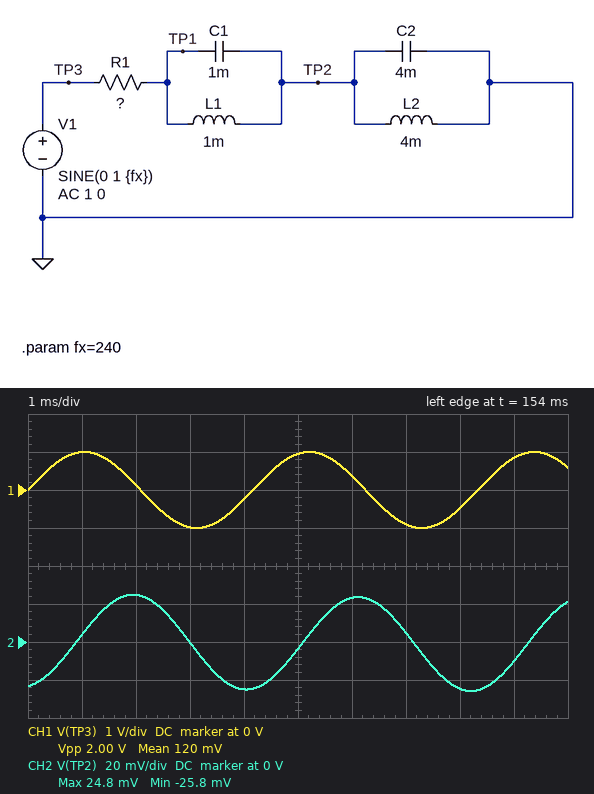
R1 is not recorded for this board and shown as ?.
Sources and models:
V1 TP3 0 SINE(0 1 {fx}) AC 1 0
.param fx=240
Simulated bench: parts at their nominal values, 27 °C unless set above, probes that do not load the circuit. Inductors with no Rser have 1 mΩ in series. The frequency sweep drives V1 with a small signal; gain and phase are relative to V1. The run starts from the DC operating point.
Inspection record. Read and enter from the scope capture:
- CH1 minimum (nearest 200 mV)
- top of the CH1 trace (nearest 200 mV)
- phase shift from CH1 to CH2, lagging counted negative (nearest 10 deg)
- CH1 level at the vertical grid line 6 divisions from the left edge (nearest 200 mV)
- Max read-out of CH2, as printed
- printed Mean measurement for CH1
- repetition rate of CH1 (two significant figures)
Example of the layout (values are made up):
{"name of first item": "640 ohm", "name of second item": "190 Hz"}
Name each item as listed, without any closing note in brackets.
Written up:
{"CH1 minimum": "-1.0 V", "top of the CH1 trace": "1.0 V", "phase shift from CH1 to CH2, lagging counted negative": "-80 deg", "CH1 level at the vertical grid line 6 divisions from the left edge": "400 mV", "Max read-out of CH2, as printed": "24.8 mV", "printed Mean measurement for CH1": "120 mV", "repetition rate of CH1": "240 Hz"}
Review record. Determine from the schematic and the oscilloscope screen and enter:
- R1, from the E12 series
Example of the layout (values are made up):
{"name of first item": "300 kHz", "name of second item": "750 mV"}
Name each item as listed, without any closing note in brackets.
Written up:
{"R1, from the E12 series": "6.8 Ω"}
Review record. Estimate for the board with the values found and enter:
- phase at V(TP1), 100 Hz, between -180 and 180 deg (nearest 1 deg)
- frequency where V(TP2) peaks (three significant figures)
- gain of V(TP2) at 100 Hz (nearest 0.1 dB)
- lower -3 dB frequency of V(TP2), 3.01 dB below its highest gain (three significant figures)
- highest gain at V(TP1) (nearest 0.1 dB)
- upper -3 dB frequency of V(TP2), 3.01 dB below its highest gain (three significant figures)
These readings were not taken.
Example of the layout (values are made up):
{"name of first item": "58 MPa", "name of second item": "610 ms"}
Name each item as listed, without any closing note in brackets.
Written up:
{"phase at V(TP1), 100 Hz, between -180 and 180 deg": "85 deg", "frequency where V(TP2) peaks": "39.9 Hz", "gain of V(TP2) at 100 Hz": "-23.2 dB", "lower -3 dB frequency of V(TP2), 3.01 dB below its highest gain": "37.1 Hz", "highest gain at V(TP1)": "-0.1 dB", "upper -3 dB frequency of V(TP2), 3.01 dB below its highest gain": "43.0 Hz"}
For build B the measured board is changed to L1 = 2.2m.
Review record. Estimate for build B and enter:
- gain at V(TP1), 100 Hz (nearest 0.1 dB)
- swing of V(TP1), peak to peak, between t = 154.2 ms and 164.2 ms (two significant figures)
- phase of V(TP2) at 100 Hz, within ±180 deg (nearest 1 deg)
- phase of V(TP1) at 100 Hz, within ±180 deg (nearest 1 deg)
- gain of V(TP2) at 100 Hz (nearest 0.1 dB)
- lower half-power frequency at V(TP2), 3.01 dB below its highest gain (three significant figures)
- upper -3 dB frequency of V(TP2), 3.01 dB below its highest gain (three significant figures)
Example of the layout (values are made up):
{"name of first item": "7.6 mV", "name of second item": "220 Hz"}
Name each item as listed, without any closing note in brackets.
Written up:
{"gain at V(TP1), 100 Hz": "-1.7 dB", "swing of V(TP1), peak to peak, between t = 154.2 ms and 164.2 ms": "290 mV", "phase of V(TP2) at 100 Hz, within ±180 deg": "-146 deg", "phase of V(TP1) at 100 Hz, within ±180 deg": "34 deg", "gain of V(TP2) at 100 Hz": "-28.2 dB", "lower half-power frequency at V(TP2), 3.01 dB below its highest gain": "37.2 Hz", "upper -3 dB frequency of V(TP2), 3.01 dB below its highest gain": "43.1 Hz"}
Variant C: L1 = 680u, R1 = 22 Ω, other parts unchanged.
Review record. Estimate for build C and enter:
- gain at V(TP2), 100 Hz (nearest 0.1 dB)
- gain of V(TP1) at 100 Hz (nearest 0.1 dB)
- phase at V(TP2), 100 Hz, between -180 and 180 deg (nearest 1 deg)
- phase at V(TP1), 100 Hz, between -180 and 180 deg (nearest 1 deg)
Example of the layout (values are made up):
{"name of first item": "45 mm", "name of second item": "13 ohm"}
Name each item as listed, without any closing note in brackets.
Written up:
{"gain at V(TP2), 100 Hz": "-33.4 dB", "gain of V(TP1) at 100 Hz": "-45.9 dB", "phase at V(TP2), 100 Hz, between -180 and 180 deg": "-90 deg", "phase at V(TP1), 100 Hz, between -180 and 180 deg": "89 deg"}
